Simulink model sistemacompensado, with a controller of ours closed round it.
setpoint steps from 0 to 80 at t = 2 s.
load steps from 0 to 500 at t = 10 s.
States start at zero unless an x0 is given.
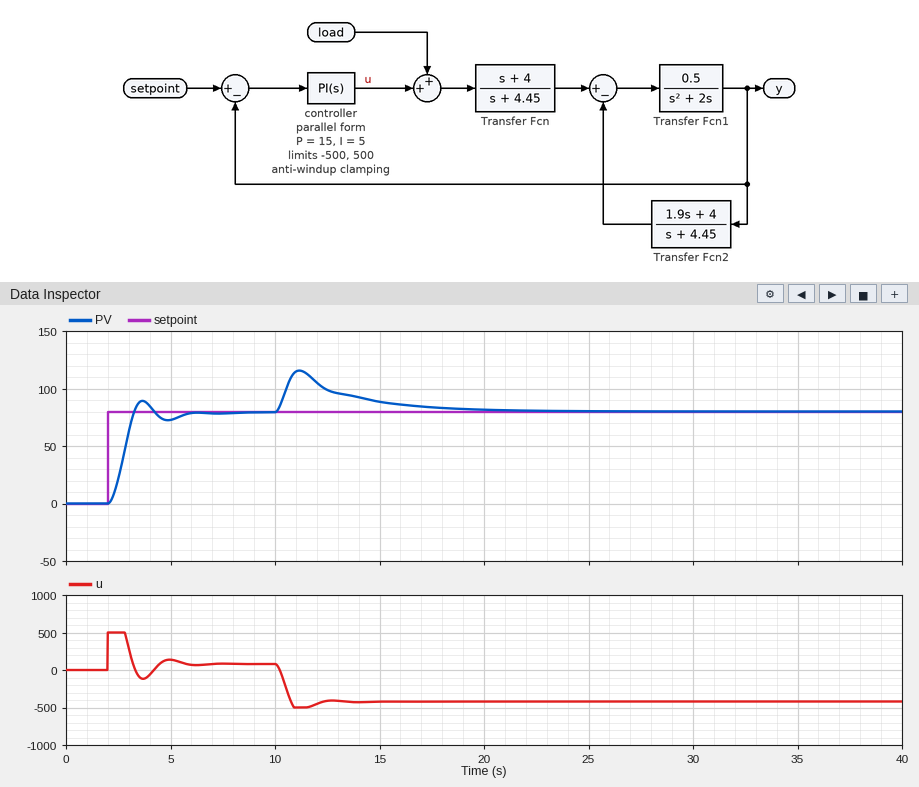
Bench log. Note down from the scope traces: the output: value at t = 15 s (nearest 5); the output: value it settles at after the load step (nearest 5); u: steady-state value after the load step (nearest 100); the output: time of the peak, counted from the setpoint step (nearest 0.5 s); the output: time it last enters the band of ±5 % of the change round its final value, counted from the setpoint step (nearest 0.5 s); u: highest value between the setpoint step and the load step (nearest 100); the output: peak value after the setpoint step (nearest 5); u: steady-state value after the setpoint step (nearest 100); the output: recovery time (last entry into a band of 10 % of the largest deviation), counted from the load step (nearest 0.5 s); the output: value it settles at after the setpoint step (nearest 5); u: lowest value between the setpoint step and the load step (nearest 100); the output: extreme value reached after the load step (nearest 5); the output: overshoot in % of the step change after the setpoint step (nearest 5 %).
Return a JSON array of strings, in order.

["90", "80", "-400", "1.5 s", "3.5 s", "500", "90", "100", "7.5 s", "80", "-100", "115", "10 %"]
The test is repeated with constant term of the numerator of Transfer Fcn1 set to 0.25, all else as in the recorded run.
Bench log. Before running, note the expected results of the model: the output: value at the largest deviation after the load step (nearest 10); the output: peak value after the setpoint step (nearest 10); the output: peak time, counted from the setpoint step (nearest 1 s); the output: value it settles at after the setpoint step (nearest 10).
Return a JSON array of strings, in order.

["110", "80", "3 s", "80"]
